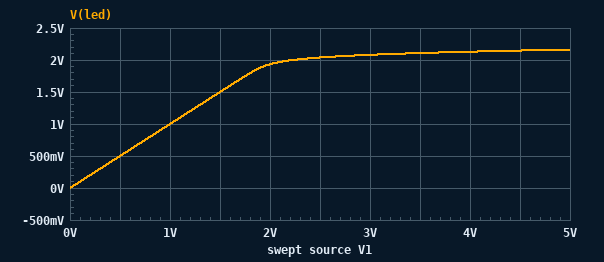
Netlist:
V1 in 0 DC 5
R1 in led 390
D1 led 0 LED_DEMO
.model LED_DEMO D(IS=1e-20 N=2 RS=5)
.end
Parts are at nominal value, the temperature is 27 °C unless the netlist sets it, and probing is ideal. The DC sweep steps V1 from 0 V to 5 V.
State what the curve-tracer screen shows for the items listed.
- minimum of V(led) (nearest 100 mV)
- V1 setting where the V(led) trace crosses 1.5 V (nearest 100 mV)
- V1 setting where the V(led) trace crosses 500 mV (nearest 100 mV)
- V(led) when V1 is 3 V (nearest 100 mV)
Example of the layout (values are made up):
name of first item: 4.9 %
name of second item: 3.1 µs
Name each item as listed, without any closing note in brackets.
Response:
minimum of V(led): 0 V
V1 setting where the V(led) trace crosses 1.5 V: 1.5 V
V1 setting where the V(led) trace crosses 500 mV: 500 mV
V(led) when V1 is 3 V: 2.1 V
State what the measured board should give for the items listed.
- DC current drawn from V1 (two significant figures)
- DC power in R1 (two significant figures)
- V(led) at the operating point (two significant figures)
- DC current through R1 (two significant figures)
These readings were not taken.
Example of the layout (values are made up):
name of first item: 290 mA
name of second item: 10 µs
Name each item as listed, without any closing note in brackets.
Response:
DC current drawn from V1: 7.3 mA
DC power in R1: 21 mW
V(led) at the operating point: 2.2 V
DC current through R1: 7.3 mA
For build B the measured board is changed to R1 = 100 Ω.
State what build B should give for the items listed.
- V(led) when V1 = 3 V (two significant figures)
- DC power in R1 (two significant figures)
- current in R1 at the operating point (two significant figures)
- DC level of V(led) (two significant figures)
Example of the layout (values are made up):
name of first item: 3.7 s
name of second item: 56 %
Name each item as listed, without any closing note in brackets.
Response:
V(led) when V1 = 3 V: 2.2 V
DC power in R1: 71 mW
current in R1 at the operating point: 27 mA
DC level of V(led): 2.3 V
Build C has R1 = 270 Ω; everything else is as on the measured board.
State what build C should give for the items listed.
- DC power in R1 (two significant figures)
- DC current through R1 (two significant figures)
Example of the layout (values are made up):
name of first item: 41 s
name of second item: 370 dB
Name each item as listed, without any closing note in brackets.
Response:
DC power in R1: 29 mW
DC current through R1: 10 mA
